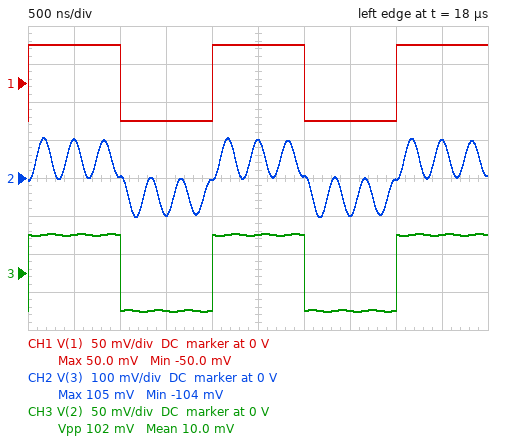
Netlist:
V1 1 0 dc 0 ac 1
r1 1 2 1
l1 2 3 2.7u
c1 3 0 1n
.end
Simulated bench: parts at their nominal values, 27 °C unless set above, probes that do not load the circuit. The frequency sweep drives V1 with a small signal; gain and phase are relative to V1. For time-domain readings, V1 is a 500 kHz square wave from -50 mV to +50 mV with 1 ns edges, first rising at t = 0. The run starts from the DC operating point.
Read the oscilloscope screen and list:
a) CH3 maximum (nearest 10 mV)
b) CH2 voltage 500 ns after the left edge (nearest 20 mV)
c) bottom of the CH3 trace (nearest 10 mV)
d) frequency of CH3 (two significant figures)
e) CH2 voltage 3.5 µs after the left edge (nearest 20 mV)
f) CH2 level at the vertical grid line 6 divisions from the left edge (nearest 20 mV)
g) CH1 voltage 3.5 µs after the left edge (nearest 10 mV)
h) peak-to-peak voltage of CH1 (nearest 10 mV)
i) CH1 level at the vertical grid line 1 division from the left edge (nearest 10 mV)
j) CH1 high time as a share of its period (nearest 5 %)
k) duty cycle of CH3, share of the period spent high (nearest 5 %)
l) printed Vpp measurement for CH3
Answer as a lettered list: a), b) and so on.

a) 50 mV
b) 100 mV
c) -50 mV
d) 500 kHz
e) -100 mV
f) 0 V
g) -50 mV
h) 100 mV
i) 50 mV
j) 50 %
k) 50 %
l) 102 mV
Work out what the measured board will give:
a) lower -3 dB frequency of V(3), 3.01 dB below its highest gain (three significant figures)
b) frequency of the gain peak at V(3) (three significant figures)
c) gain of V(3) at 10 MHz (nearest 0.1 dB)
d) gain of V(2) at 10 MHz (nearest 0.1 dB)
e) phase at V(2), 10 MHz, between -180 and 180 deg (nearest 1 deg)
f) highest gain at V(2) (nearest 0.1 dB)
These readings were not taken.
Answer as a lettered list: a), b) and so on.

a) 3.03 MHz
b) 3.06 MHz
c) -19.7 dB
d) 0 dB
e) 0 deg
f) 0 dB
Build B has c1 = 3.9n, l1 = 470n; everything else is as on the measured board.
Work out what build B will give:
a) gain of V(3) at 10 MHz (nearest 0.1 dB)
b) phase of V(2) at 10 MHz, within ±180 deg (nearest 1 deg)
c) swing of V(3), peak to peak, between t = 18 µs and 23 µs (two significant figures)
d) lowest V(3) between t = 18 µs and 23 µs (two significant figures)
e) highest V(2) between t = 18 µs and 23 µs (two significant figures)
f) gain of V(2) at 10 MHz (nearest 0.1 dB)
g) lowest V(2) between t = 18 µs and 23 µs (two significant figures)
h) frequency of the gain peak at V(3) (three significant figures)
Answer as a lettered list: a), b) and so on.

a) -15.9 dB
b) 2 deg
c) 280 mV
d) -140 mV
e) 58 mV
f) 0 dB
g) -58 mV
h) 3.71 MHz
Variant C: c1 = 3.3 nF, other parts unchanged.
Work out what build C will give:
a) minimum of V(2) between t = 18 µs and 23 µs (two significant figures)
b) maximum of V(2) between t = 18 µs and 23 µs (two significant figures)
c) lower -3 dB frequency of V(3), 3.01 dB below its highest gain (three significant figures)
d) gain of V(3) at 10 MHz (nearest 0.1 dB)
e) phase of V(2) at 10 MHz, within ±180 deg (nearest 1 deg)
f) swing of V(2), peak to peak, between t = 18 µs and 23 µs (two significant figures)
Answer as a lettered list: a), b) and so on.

a) -53 mV
b) 53 mV
c) 1.66 MHz
d) -30.7 dB
e) 0 deg
f) 110 mV
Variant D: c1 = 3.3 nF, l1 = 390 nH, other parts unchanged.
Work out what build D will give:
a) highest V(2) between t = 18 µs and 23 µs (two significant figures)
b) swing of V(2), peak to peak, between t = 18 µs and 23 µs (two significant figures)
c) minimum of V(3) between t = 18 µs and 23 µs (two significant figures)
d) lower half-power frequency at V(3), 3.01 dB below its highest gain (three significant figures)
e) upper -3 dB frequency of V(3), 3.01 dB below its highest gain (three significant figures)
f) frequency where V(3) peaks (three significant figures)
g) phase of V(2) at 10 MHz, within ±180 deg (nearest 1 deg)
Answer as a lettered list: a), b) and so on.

a) 60 mV
b) 120 mV
c) -160 mV
d) 4.22 MHz
e) 4.63 MHz
f) 4.43 MHz
g) 3 deg
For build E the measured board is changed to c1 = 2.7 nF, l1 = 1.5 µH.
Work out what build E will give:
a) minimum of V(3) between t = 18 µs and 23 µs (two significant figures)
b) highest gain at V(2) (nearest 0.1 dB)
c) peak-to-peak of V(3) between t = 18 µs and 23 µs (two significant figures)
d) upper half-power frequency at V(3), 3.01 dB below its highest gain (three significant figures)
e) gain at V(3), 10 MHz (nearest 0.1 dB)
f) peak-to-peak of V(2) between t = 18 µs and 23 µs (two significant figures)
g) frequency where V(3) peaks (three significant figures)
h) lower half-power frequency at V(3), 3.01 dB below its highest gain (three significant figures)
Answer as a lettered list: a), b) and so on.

a) -380 mV
b) 0 dB
c) 760 mV
d) 2.55 MHz
e) -23.5 dB
f) 130 mV
g) 2.50 MHz
h) 2.45 MHz
